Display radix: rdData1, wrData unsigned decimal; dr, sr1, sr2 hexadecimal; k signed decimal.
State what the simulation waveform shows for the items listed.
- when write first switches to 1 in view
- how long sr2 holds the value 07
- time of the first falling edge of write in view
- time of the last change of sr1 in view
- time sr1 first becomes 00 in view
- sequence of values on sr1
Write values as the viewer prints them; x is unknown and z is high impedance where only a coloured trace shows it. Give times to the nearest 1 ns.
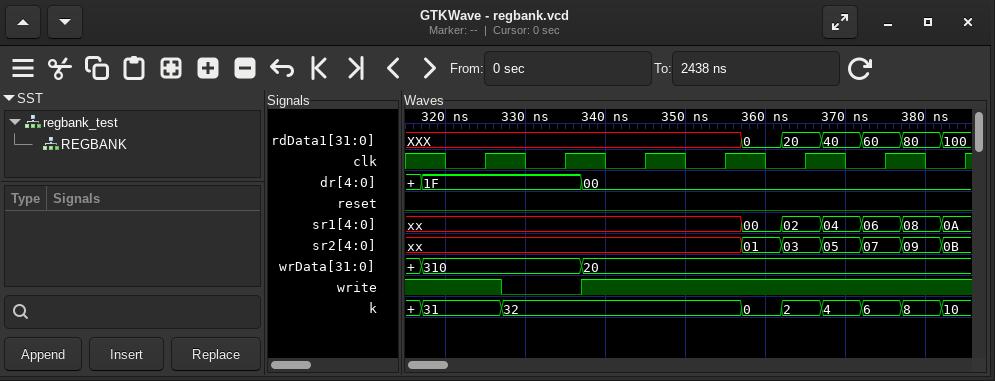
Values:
337 ns
5 ns
327 ns
382 ns
357 ns
xx, 00, 02, 04, 06, 08, 0A
